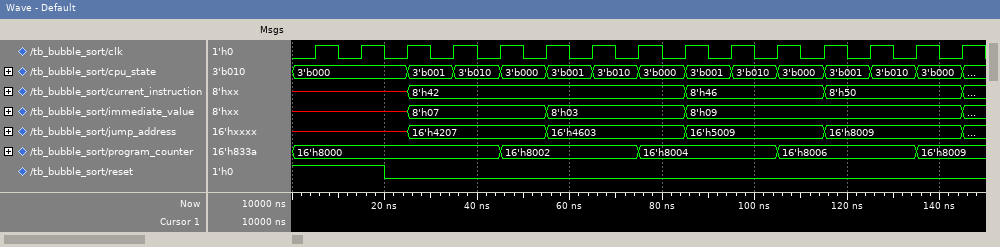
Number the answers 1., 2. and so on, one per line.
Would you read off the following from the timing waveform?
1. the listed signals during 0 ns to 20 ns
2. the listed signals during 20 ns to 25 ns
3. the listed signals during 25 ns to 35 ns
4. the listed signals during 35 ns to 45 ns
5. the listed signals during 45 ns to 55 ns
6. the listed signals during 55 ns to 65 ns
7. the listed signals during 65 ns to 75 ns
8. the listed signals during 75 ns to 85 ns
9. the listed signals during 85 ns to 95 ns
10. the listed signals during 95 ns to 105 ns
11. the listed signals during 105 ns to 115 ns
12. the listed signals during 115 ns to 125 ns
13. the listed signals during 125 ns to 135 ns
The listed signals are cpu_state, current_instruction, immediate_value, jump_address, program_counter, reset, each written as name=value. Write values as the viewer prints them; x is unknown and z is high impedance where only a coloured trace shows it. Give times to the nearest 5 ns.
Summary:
1. cpu_state=3'b000, current_instruction=x, immediate_value=x, jump_address=x, program_counter=16'h8000, reset=1
2. cpu_state=3'b000, current_instruction=x, immediate_value=x, jump_address=x, program_counter=16'h8000, reset=0
3. cpu_state=3'b001, current_instruction=8'h42, immediate_value=8'h07, jump_address=16'h4207, program_counter=16'h8000, reset=0
4. cpu_state=3'b010, current_instruction=8'h42, immediate_value=8'h07, jump_address=16'h4207, program_counter=16'h8000, reset=0
5. cpu_state=3'b000, current_instruction=8'h42, immediate_value=8'h07, jump_address=16'h4207, program_counter=16'h8002, reset=0
6. cpu_state=3'b001, current_instruction=8'h42, immediate_value=8'h03, jump_address=16'h4603, program_counter=16'h8002, reset=0
7. cpu_state=3'b010, current_instruction=8'h42, immediate_value=8'h03, jump_address=16'h4603, program_counter=16'h8002, reset=0
8. cpu_state=3'b000, current_instruction=8'h42, immediate_value=8'h03, jump_address=16'h4603, program_counter=16'h8004, reset=0
9. cpu_state=3'b001, current_instruction=8'h46, immediate_value=8'h09, jump_address=16'h5009, program_counter=16'h8004, reset=0
10. cpu_state=3'b010, current_instruction=8'h46, immediate_value=8'h09, jump_address=16'h5009, program_counter=16'h8004, reset=0
11. cpu_state=3'b000, current_instruction=8'h46, immediate_value=8'h09, jump_address=16'h5009, program_counter=16'h8006, reset=0
12. cpu_state=3'b001, current_instruction=8'h50, immediate_value=8'h09, jump_address=16'h8009, program_counter=16'h8006, reset=0
13. cpu_state=3'b010, current_instruction=8'h50, immediate_value=8'h09, jump_address=16'h8009, program_counter=16'h8006, reset=0
